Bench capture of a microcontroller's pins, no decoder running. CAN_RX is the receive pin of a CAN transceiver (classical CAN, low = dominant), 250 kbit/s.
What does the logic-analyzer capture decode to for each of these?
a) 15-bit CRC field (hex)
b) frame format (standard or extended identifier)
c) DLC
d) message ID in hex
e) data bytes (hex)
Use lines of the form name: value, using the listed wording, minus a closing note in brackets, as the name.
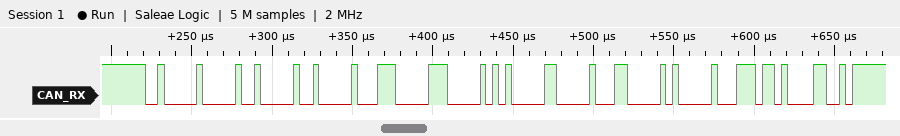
15-bit CRC field: 0x6D0C
frame format: standard
DLC: 8
message ID in hex: 0x200
data bytes: 08 07 06 05 04 03 02 01
